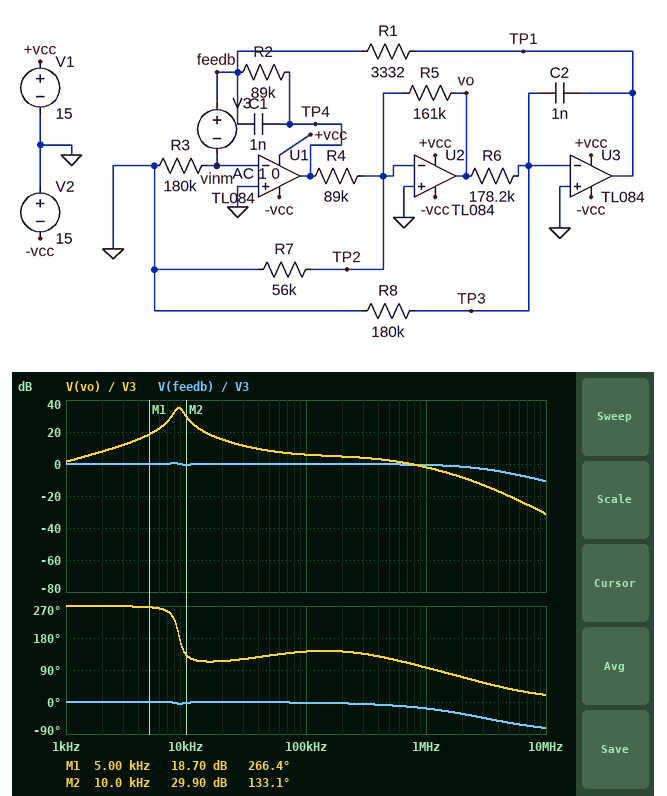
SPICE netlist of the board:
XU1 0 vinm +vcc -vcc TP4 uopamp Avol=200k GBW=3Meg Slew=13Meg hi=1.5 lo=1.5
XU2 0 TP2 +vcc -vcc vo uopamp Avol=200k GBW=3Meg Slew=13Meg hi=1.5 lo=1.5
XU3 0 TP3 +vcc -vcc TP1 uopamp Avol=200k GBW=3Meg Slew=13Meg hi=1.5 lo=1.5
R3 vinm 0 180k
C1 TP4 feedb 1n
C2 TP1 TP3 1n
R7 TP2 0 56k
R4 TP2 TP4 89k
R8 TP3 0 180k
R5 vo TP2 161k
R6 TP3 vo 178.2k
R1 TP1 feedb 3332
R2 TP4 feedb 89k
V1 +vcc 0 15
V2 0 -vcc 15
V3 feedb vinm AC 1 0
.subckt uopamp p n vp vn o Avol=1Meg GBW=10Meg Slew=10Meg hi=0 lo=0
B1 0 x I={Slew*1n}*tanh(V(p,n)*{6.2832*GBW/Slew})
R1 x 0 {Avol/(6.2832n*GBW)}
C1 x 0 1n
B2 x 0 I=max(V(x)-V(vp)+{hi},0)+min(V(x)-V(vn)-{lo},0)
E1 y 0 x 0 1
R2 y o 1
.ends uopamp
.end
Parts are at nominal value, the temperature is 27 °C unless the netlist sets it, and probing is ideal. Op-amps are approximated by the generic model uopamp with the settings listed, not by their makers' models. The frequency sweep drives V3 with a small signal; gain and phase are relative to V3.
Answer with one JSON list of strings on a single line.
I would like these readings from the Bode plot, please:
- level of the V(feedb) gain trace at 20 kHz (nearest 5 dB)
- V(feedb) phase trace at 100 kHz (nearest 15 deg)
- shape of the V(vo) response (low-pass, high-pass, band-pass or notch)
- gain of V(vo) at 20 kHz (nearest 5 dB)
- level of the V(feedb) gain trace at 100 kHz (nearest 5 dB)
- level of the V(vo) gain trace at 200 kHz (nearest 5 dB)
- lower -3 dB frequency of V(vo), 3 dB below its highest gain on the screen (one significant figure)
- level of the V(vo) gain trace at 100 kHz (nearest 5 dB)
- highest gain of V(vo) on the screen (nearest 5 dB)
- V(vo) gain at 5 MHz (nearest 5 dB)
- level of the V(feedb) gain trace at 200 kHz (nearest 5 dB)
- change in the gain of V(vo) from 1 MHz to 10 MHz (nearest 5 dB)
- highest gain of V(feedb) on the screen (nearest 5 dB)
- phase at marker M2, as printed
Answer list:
["0 dB", "0 deg", "band-pass", "15 dB", "0 dB", "5 dB", "8 kHz", "5 dB", "35 dB", "-20 dB", "0 dB", "-30 dB", "0 dB", "133.1 deg"]
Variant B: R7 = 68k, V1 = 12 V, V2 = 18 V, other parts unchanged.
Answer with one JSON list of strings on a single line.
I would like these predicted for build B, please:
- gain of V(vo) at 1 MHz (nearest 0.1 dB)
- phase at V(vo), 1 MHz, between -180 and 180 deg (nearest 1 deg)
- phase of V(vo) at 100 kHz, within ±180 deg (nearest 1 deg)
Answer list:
["-1.4 dB", "99 deg", "143 deg"]
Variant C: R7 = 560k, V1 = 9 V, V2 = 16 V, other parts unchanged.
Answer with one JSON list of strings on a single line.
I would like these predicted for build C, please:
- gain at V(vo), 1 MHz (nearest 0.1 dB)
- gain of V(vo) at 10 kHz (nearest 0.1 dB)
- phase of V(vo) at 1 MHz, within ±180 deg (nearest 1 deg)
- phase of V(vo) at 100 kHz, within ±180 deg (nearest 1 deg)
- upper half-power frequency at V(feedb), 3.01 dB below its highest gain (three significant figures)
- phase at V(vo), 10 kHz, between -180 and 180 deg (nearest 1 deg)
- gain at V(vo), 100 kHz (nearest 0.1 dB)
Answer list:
["1.4 dB", "29.8 dB", "113 deg", "147 deg", "2.66 MHz", "135 deg", "6.0 dB"]
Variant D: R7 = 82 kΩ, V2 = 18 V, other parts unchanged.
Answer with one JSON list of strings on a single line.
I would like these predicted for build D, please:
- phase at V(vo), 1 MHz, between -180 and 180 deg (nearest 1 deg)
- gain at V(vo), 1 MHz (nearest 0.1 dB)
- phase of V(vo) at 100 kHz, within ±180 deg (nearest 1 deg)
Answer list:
["101 deg", "-0.9 dB", "144 deg"]
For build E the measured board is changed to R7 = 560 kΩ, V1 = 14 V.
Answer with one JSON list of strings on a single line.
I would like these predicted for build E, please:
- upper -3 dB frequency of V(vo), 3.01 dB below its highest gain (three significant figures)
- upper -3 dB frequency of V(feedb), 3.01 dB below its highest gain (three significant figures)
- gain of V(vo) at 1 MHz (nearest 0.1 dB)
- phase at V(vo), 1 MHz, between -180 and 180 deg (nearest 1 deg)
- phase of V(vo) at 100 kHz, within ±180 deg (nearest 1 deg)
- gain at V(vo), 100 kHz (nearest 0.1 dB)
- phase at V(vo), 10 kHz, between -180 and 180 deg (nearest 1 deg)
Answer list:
["9.57 kHz", "2.66 MHz", "1.4 dB", "113 deg", "147 deg", "6.0 dB", "135 deg"]
